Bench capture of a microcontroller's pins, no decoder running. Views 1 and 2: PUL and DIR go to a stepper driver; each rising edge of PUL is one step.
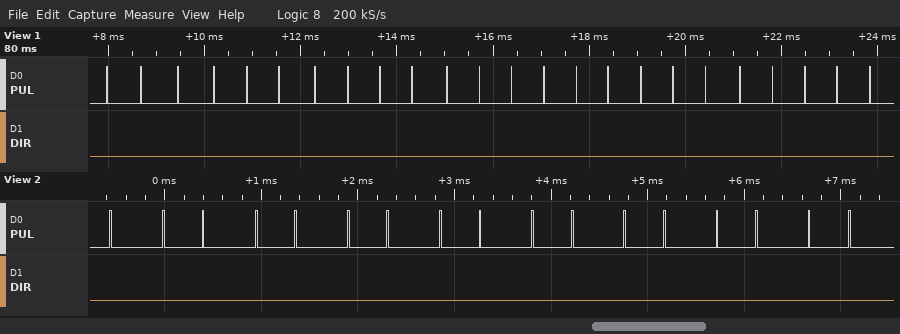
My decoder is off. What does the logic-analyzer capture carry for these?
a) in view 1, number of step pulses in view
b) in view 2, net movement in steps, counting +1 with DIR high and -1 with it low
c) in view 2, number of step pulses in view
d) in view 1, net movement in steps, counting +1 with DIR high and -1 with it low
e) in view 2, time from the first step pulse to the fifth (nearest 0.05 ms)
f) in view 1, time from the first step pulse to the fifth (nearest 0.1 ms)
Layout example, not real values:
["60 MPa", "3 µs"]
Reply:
["24", "-17", "17", "-24", "1.90 ms", "2.9 ms"]
